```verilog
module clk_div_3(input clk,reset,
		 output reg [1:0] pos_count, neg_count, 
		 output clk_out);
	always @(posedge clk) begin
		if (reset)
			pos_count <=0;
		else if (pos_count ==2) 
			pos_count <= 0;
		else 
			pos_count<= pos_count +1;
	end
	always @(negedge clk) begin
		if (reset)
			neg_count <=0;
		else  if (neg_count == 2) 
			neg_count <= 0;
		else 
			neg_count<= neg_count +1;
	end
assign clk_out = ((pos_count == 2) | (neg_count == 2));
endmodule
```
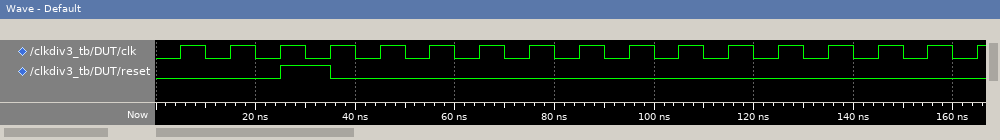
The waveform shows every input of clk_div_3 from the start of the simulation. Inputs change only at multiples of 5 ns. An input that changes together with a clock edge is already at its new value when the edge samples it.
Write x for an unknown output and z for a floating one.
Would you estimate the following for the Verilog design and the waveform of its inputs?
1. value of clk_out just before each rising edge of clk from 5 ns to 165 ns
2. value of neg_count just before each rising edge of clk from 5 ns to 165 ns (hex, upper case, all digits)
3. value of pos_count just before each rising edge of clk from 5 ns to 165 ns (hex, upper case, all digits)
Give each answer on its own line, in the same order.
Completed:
x x x 0 0 1 0 0 1 0 0 1 0 0 1 0 0
x, x, x, 0, 1, 2, 0, 1, 2, 0, 1, 2, 0, 1, 2, 0, 1
x, x, x, 0, 1, 2, 0, 1, 2, 0, 1, 2, 0, 1, 2, 0, 1
